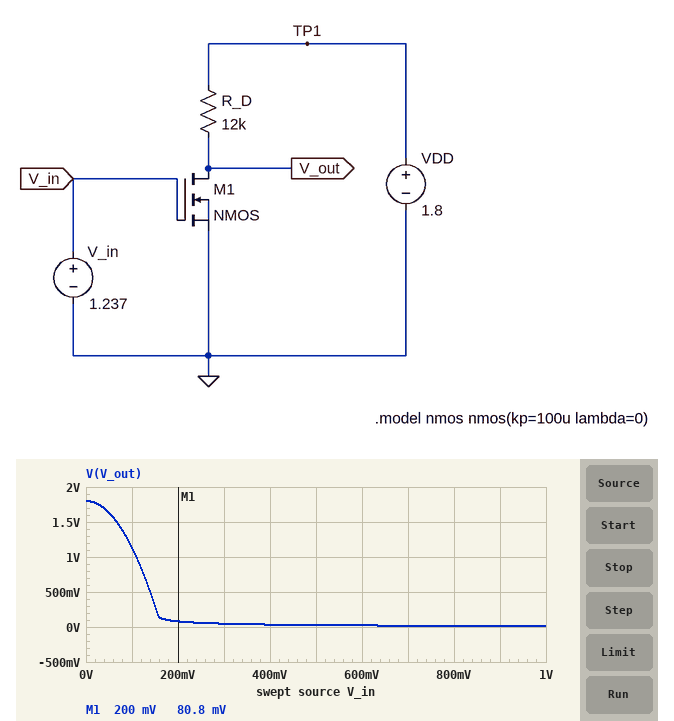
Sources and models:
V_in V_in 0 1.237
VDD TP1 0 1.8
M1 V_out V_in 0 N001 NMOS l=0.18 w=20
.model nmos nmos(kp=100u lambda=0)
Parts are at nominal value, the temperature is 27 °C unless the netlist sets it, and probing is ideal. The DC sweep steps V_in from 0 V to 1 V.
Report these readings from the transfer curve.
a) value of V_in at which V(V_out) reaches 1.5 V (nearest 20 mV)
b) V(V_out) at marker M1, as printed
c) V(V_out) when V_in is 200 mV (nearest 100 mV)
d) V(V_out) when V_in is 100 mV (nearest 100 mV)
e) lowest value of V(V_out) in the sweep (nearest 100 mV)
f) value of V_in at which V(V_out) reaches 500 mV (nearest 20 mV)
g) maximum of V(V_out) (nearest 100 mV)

60 mV
80.8 mV
100 mV
1.1 V
0 V
140 mV
1.8 V
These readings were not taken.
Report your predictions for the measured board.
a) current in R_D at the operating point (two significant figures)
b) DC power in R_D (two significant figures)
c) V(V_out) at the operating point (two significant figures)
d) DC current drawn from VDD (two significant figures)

150 µA
270 µW
11 mV
150 µA
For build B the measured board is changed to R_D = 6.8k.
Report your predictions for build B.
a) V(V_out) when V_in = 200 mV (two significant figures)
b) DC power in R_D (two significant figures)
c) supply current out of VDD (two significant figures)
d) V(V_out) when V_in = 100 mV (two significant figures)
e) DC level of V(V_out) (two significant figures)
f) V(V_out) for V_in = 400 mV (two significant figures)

290 mV
470 µW
260 µA
1.4 V
19 mV
62 mV
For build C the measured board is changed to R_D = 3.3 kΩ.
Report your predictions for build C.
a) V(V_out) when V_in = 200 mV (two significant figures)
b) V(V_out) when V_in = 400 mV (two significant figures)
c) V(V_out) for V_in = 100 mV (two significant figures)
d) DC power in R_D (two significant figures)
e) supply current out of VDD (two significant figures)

1.1 V
140 mV
1.6 V
940 µW
530 µA
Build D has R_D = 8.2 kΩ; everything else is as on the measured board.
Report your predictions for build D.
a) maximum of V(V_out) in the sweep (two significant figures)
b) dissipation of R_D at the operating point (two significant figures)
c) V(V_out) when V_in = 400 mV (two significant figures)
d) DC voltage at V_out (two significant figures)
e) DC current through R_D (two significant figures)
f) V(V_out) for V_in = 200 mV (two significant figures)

1.8 V
390 µW
51 mV
16 mV
220 µA
140 mV
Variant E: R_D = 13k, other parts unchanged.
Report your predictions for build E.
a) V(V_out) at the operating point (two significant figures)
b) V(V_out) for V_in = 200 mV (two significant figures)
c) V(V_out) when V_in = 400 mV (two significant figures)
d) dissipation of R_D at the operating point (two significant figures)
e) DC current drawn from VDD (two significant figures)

10 mV
73 mV
32 mV
250 µW
140 µA
